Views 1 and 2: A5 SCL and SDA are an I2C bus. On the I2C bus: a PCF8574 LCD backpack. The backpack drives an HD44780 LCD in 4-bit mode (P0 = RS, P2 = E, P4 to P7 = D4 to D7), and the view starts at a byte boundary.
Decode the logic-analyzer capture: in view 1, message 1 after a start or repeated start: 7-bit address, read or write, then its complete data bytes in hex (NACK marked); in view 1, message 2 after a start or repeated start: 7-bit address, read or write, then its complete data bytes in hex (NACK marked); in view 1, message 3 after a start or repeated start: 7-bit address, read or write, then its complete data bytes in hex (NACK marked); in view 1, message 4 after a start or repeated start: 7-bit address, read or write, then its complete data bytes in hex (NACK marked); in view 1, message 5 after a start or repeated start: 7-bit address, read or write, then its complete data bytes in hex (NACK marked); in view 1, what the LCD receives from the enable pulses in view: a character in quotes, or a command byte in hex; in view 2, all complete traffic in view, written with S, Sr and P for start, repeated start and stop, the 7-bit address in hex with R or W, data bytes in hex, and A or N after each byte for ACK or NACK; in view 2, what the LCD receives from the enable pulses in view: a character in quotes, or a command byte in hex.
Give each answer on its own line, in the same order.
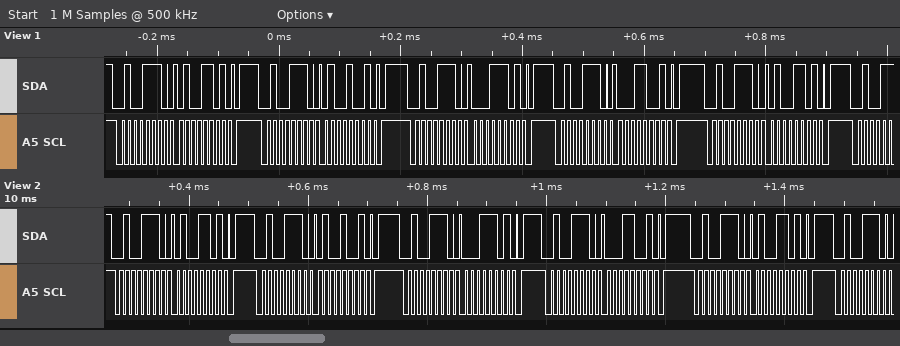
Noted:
0x27 write: 4D
0x27 write: 49
0x27 write: 1D
0x27 write: 19
0x27 write: 4D
'A'
S 27W A 4D A P S 27W A 49 A P S 27W A 1D A P S 27W A 19 A P S 27W A 4D A P S 27W A
'A'
